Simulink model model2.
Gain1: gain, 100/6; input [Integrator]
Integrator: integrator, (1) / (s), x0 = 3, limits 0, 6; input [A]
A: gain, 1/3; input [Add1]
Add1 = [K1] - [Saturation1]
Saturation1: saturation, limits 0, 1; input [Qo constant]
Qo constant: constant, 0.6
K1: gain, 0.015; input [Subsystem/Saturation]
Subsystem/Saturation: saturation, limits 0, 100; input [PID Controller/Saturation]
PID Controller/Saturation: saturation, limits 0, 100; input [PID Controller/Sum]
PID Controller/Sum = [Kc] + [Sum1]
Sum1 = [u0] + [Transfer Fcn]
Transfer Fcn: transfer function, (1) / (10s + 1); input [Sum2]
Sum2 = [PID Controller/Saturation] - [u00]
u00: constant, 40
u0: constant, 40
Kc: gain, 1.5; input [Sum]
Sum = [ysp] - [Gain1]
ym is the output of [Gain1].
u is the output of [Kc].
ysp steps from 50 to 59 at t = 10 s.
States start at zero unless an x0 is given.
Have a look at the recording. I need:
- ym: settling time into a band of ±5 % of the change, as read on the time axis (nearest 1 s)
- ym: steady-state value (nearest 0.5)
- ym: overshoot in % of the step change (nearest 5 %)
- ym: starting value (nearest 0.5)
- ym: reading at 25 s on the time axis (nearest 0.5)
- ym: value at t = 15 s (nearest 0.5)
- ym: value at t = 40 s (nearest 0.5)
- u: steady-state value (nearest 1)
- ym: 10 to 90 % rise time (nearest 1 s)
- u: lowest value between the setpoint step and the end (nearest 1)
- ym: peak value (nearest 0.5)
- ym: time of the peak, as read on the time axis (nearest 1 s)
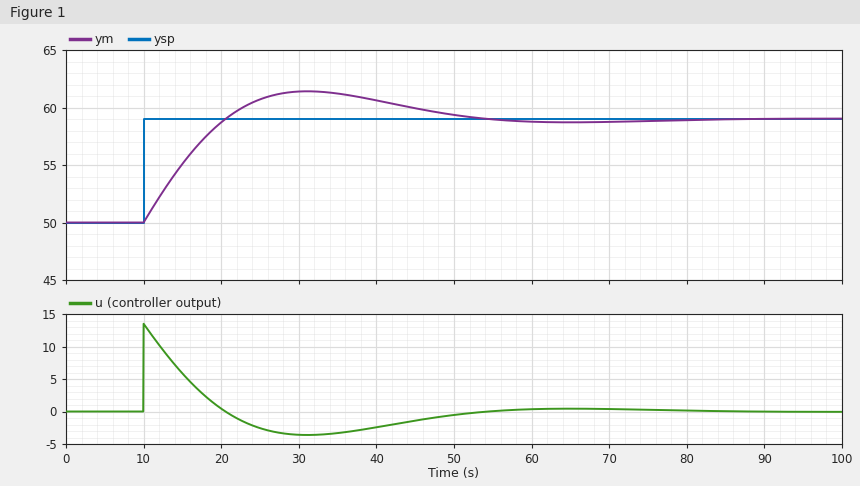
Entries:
49 s
59.0
25 %
50.0
60.5
55.0
60.5
0
8 s
-4
61.5
31 s
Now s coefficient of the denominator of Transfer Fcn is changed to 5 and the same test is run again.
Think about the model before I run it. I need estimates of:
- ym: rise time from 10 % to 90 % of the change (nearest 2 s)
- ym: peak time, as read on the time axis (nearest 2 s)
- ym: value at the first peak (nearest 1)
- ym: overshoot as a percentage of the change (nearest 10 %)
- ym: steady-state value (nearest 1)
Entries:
6 s
26 s
62
40 %
59
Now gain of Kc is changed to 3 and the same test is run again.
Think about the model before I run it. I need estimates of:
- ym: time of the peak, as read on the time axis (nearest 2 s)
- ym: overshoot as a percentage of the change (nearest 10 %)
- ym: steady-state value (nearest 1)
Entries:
24 s
20 %
59
